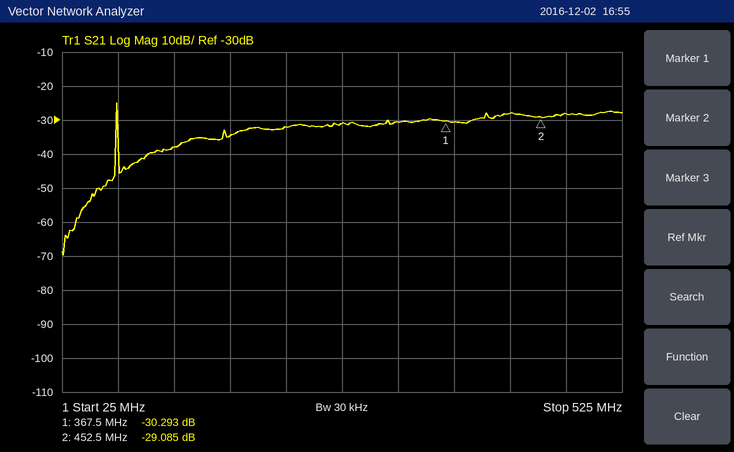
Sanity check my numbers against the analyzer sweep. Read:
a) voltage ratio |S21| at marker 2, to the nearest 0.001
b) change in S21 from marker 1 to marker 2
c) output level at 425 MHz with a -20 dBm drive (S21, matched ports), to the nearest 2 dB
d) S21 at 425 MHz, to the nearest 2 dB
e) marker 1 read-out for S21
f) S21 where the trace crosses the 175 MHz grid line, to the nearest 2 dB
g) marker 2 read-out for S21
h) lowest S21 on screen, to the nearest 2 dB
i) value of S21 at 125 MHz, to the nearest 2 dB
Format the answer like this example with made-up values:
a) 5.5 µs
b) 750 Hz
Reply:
a) 0.035
b) 1.208 dB
c) -48 dBm
d) -28 dB
e) -30.293 dB
f) -34 dB
g) -29.085 dB
h) -70 dB
i) -38 dB
